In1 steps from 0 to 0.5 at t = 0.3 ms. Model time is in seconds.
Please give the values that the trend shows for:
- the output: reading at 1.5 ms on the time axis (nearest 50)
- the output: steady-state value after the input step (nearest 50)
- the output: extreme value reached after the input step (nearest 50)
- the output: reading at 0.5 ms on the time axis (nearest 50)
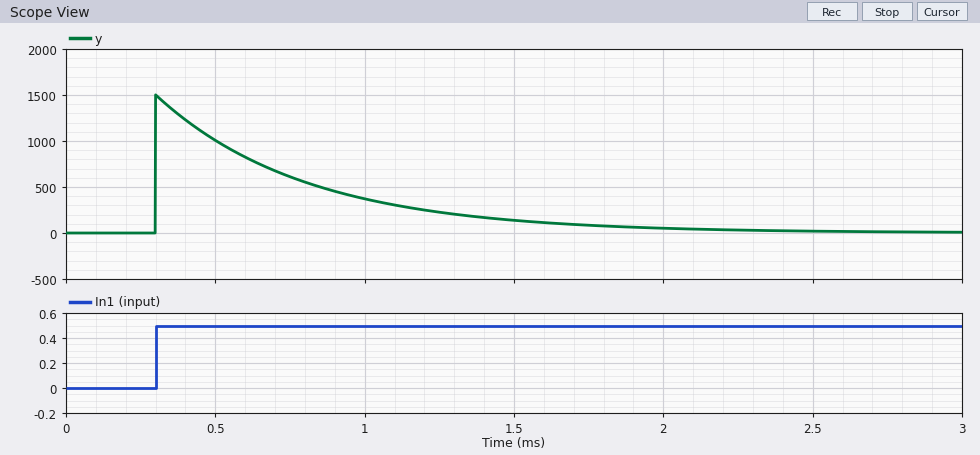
150
0
1500
1000
